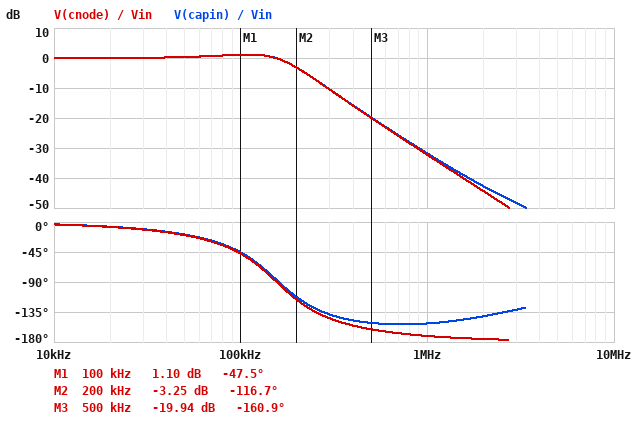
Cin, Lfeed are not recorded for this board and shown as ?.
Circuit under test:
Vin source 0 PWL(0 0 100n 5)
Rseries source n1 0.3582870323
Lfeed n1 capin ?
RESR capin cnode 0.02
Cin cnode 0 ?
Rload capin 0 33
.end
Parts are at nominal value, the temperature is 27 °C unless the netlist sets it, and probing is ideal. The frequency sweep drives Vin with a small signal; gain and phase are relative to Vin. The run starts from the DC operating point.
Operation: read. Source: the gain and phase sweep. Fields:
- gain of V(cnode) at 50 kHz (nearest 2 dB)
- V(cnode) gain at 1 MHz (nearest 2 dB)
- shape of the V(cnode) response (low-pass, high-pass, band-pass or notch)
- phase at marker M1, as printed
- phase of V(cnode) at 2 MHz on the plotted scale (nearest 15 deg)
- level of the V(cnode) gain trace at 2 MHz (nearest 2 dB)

0 dB
-32 dB
low-pass
-47.5 deg
-180 deg
-44 dB
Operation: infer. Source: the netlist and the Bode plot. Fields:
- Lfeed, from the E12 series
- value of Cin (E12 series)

390 nH
2.7 µF
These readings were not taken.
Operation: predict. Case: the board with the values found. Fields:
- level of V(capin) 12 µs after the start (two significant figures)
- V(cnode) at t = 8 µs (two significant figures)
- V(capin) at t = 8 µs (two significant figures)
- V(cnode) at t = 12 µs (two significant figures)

5.0 V
4.8 V
4.8 V
5.0 V
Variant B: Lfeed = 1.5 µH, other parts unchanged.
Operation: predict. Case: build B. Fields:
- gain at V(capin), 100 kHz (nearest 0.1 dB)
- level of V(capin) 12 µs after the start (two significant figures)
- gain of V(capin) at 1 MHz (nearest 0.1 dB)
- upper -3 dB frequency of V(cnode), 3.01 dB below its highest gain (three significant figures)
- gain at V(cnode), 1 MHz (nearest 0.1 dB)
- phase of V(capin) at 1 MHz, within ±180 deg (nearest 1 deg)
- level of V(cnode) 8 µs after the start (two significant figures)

1.0 dB
4.2 V
-43.6 dB
93.0 kHz
-44.0 dB
-159 deg
6.6 V
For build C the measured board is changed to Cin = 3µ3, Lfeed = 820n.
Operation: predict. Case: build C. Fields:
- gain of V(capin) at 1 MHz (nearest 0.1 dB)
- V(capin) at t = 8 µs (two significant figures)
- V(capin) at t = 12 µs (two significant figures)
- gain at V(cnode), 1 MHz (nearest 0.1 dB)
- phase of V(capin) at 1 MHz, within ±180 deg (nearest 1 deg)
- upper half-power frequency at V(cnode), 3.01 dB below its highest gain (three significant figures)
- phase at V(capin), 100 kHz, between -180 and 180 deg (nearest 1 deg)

-39.8 dB
5.4 V
4.6 V
-40.5 dB
-153 deg
116 kHz
-92 deg
